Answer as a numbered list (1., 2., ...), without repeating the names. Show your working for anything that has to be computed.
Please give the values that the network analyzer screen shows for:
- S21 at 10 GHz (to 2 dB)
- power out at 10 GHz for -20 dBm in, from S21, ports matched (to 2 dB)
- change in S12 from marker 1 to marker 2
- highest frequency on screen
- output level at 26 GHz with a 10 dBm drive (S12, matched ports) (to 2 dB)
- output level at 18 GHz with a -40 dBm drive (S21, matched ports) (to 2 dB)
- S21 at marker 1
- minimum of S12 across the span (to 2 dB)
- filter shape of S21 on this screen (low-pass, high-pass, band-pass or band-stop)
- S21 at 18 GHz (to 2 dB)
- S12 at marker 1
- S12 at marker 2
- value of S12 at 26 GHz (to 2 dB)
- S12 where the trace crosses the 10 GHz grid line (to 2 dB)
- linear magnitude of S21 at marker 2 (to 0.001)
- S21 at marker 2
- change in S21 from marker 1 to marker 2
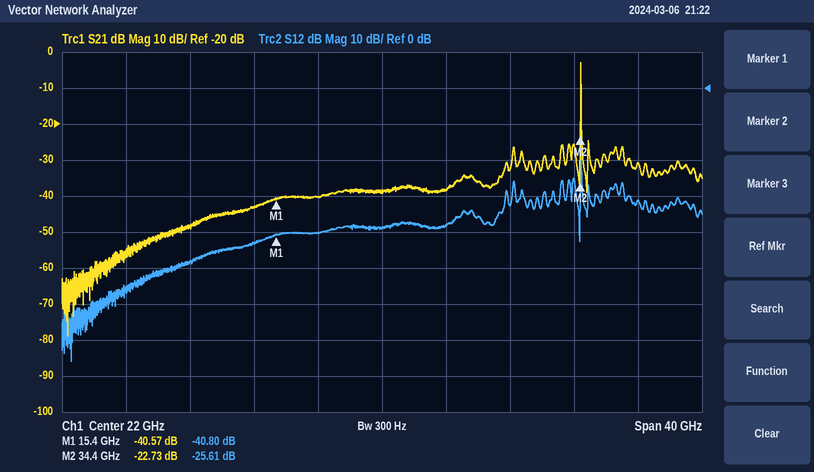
1. -48 dB
2. -20 dBm + (-48 dB) = -68 dBm
3. -25.61 − (-40.8) = 15.19 dB
4. 42 GHz
5. 10 dBm + (-38 dB) = -28 dBm
6. -40 dBm + (-40 dB) = -80 dBm
7. -40.57 dB
8. -76 dB
9. band-pass
10. -40 dB
11. -40.80 dB
12. -25.61 dB
13. -38 dB
14. -48 dB
15. 10^(-22.73/20) ≈ 0.073
16. -22.73 dB
17. -22.73 − (-40.57) = 17.84 dB
